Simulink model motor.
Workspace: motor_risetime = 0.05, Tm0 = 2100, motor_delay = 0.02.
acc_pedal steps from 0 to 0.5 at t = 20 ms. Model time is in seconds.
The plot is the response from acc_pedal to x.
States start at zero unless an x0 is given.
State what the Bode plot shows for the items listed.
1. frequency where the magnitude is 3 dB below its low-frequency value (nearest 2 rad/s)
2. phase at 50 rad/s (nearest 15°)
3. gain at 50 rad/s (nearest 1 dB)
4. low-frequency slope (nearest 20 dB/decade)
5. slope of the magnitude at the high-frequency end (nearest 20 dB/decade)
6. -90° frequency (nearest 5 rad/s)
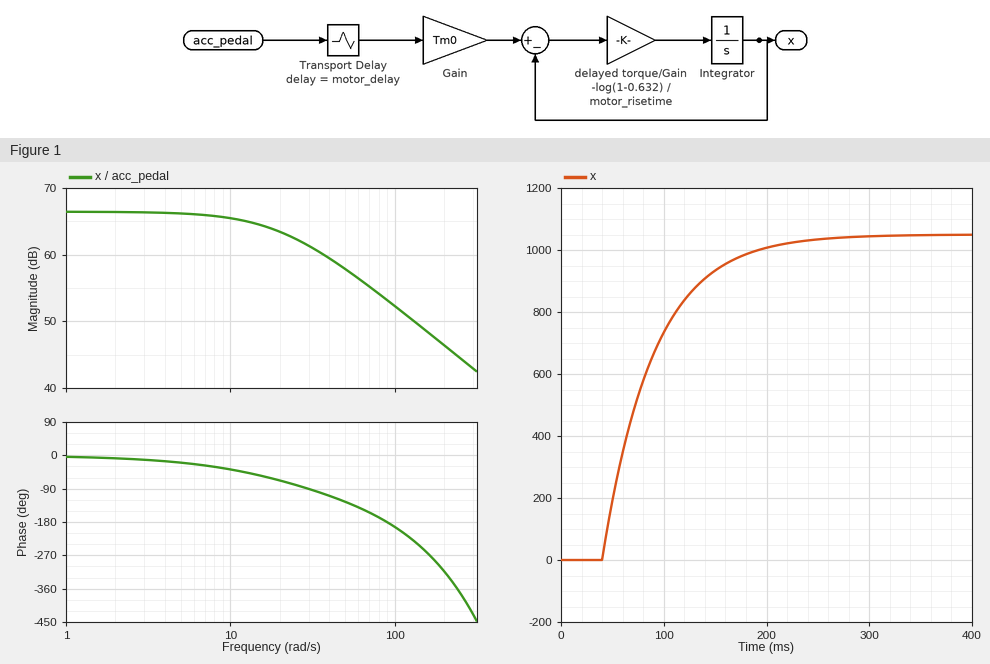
20 rad/s
-120°
58 dB
0 dB/decade
-20 dB/decade
30 rad/s
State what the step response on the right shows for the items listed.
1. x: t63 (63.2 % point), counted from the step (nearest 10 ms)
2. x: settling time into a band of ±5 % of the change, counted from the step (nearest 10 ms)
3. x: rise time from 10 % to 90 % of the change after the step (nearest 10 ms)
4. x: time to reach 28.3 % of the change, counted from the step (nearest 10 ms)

70 ms
170 ms
110 ms
40 ms
